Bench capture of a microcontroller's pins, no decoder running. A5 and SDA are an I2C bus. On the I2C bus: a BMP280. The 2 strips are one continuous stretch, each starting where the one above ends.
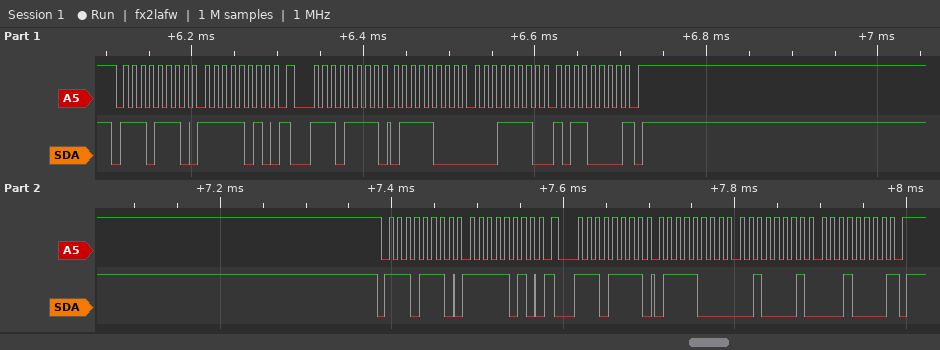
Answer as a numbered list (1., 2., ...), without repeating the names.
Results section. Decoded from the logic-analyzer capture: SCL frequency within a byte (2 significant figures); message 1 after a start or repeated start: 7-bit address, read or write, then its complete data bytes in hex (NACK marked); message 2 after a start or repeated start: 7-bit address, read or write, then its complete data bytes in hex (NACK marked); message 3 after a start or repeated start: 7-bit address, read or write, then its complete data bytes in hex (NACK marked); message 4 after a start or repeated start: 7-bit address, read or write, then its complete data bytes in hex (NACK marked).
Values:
1. 100 kHz
2. 0x77 write: FA
3. 0x77 read: 78 1E B0 NACK
4. 0x77 write: FA
5. 0x77 read: 78 21 10 NACK
